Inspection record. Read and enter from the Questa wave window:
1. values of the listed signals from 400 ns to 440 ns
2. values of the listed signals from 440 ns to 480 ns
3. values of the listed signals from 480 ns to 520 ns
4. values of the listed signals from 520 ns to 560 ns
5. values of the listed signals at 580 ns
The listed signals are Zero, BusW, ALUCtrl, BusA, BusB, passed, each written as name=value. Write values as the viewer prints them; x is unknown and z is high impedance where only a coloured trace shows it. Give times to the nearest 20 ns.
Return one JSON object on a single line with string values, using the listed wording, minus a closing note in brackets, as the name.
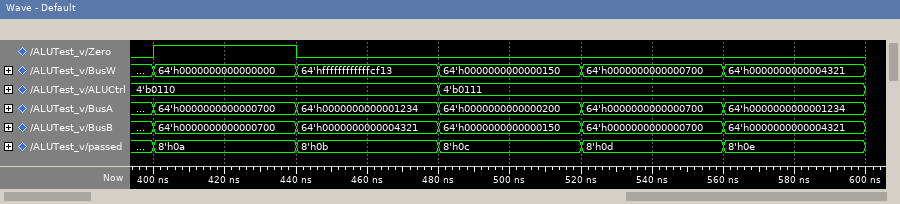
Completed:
{"values of the listed signals from 400 ns to 440 ns": "Zero=1, BusW=64'h0000000000000000, ALUCtrl=4'b0110, BusA=64'h0000000000000700, BusB=64'h0000000000000700, passed=8'h0a", "values of the listed signals from 440 ns to 480 ns": "Zero=0, BusW=64'hffffffffffffcf13, ALUCtrl=4'b0110, BusA=64'h0000000000001234, BusB=64'h0000000000004321, passed=8'h0b", "values of the listed signals from 480 ns to 520 ns": "Zero=0, BusW=64'h0000000000000150, ALUCtrl=4'b0111, BusA=64'h0000000000000200, BusB=64'h0000000000000150, passed=8'h0c", "values of the listed signals from 520 ns to 560 ns": "Zero=0, BusW=64'h0000000000000700, ALUCtrl=4'b0111, BusA=64'h0000000000000700, BusB=64'h0000000000000700, passed=8'h0d", "values of the listed signals at 580 ns": "Zero=0, BusW=64'h0000000000004321, ALUCtrl=4'b0111, BusA=64'h0000000000001234, BusB=64'h0000000000004321, passed=8'h0e"}
